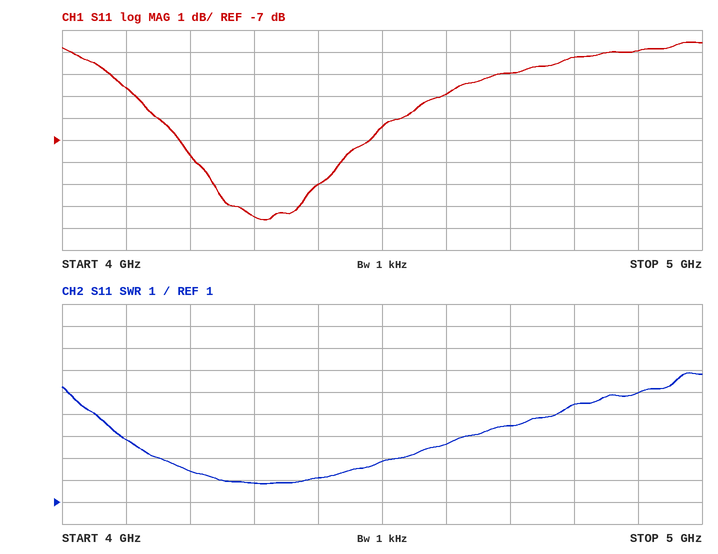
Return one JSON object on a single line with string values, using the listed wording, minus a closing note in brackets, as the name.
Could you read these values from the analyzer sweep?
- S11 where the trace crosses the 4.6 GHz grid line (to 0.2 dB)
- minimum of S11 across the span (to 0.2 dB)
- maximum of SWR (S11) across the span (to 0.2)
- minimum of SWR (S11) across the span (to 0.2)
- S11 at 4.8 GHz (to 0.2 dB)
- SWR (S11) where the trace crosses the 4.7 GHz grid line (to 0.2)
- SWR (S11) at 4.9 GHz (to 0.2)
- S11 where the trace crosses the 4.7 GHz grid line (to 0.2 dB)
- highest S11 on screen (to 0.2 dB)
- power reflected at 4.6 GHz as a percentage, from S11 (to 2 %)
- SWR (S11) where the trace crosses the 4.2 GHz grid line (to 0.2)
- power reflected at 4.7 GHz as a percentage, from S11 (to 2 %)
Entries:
{"S11 where the trace crosses the 4.6 GHz grid line": "-5.0 dB", "minimum of S11 across the span": "-10.6 dB", "maximum of SWR (S11) across the span": "6.8", "minimum of SWR (S11) across the span": "1.8", "S11 at 4.8 GHz": "-3.2 dB", "SWR (S11) where the trace crosses the 4.7 GHz grid line": "4.4", "SWR (S11) at 4.9 GHz": "6.0", "S11 where the trace crosses the 4.7 GHz grid line": "-4.0 dB", "highest S11 on screen": "-2.6 dB", "power reflected at 4.6 GHz as a percentage, from S11": "32 %", "SWR (S11) where the trace crosses the 4.2 GHz grid line": "2.4", "power reflected at 4.7 GHz as a percentage, from S11": "40 %"}
